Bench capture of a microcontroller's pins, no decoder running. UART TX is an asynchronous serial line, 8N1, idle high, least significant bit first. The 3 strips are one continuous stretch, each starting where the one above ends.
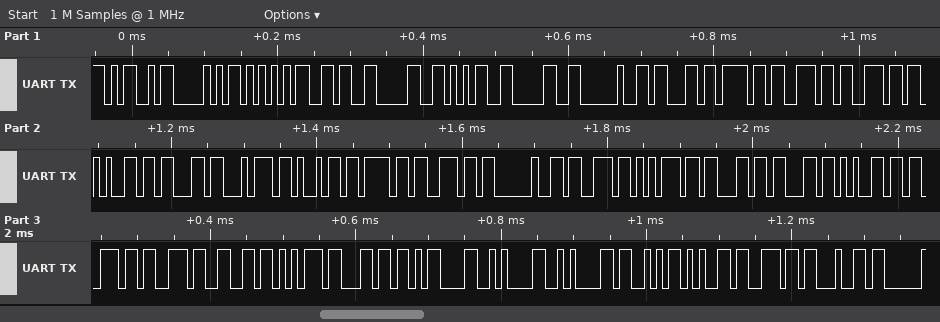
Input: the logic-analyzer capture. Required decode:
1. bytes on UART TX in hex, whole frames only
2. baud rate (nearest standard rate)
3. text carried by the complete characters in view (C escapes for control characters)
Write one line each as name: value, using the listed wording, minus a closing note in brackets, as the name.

bytes on UART TX in hex, whole frames only: 4D 50 55 36 30 35 30 20 63 6F 6E 6E 65 63 74 69 6F 6E 20 73 75 63 63 65 73 73 66 75 6C 0D 0A 0A 53 65 6E 64
baud rate: 115200 baud
text carried by the complete characters in view: "MPU6050 connection successful\r\n\nSend"
